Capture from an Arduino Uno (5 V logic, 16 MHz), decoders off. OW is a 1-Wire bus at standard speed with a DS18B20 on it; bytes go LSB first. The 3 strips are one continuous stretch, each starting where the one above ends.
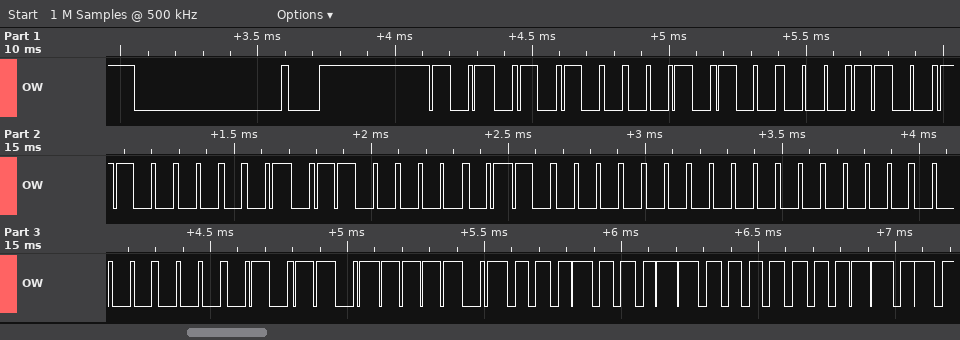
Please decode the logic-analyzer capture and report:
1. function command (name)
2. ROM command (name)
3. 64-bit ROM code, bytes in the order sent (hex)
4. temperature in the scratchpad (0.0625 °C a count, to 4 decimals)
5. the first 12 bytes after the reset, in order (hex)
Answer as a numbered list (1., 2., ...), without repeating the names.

1. Read Scratchpad
2. Match ROM
3. 28 98 81 06 06 00 00 D0
4. 24.5000 °C
5. 55 28 98 81 06 06 00 00 D0 BE 88 01
